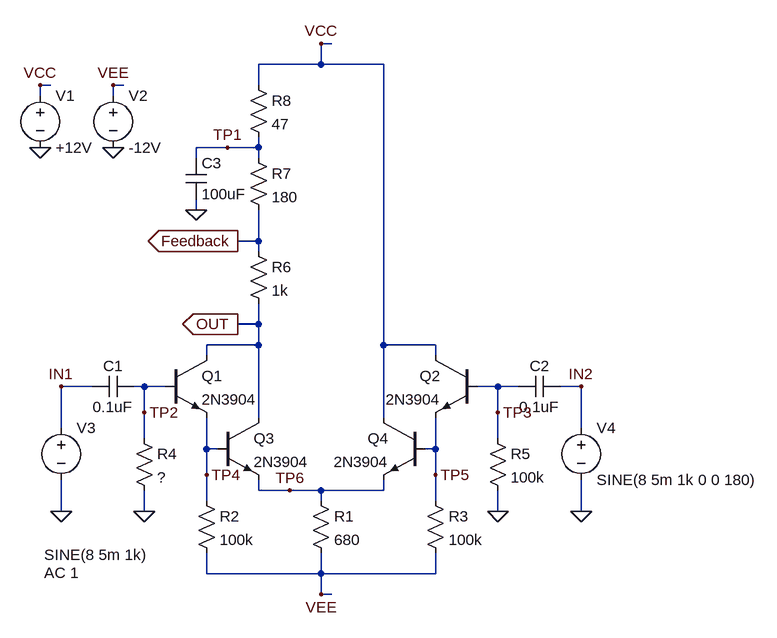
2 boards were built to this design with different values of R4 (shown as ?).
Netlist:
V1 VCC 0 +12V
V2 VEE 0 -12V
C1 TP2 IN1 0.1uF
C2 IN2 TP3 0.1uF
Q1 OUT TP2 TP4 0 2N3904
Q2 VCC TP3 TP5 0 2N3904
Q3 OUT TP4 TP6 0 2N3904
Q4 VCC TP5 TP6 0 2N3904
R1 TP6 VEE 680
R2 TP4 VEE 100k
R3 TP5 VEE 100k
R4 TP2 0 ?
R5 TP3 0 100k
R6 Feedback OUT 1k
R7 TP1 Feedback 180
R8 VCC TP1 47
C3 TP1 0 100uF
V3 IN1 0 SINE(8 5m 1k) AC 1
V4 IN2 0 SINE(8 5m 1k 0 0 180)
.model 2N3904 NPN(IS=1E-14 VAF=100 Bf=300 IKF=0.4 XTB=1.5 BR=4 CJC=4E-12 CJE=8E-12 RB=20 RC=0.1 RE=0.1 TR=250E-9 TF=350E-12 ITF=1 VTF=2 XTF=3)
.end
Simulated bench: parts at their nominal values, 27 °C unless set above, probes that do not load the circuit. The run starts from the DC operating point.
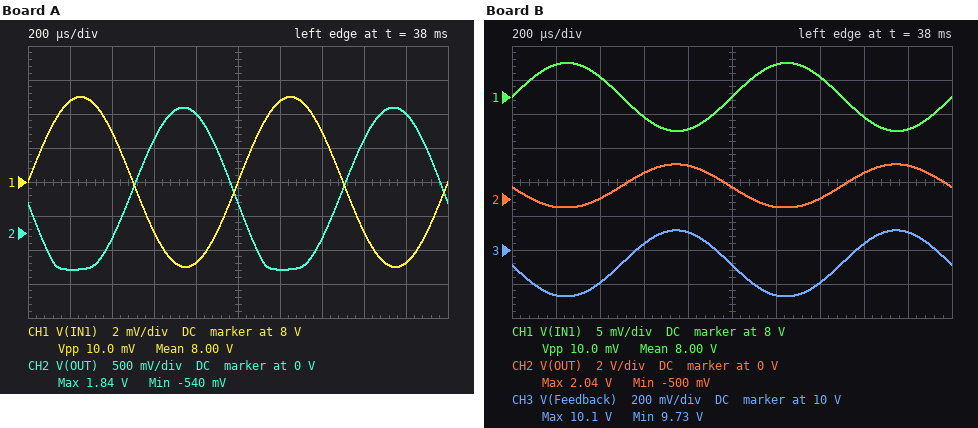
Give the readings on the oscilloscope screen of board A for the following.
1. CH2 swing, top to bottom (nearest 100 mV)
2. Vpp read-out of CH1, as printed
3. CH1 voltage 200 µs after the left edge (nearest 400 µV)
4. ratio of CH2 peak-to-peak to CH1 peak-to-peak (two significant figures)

2.4 V
10.0 mV
8.0048 V
240
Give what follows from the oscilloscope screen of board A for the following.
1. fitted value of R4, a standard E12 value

33 kΩ
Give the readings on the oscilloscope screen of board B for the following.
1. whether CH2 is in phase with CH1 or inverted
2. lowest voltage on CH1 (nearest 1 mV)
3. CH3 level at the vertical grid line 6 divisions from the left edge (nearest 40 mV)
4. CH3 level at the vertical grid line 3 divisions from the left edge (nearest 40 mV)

inverted
7.995 V
9.72 V
10.04 V
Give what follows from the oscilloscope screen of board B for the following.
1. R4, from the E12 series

47 kΩ
